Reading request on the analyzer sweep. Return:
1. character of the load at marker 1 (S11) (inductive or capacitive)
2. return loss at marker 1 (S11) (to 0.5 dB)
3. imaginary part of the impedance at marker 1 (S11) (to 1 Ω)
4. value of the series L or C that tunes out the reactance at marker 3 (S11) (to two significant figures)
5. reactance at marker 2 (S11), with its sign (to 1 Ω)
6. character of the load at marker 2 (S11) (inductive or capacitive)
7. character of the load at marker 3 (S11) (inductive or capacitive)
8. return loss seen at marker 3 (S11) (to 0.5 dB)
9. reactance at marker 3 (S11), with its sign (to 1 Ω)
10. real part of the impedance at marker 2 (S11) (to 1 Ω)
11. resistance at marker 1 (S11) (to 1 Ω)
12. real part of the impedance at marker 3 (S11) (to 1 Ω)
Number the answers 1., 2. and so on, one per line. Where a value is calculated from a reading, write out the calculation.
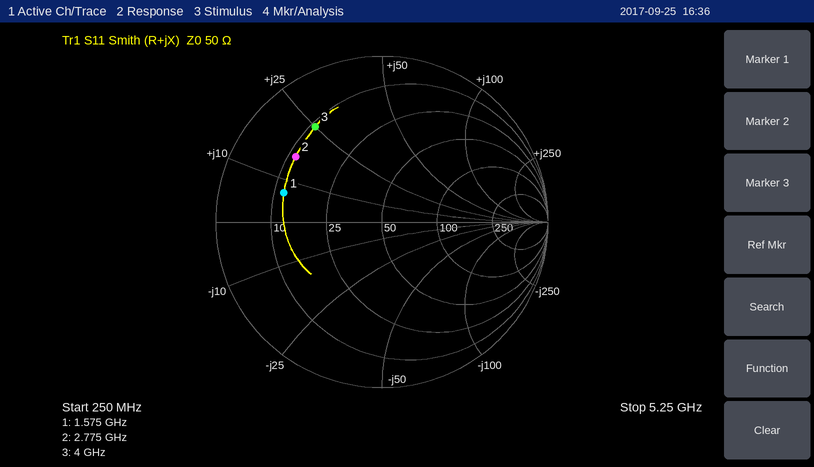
1. inductive
2. 4.0 dB
3. +7 Ω
4. C = 1/(2π × 4 GHz × 25 Ω) ≈ 1.6 pF
5. +16 Ω
6. inductive
7. inductive
8. 3.0 dB
9. +25 Ω
10. 12 Ω
11. 12 Ω
12. 11 Ω
